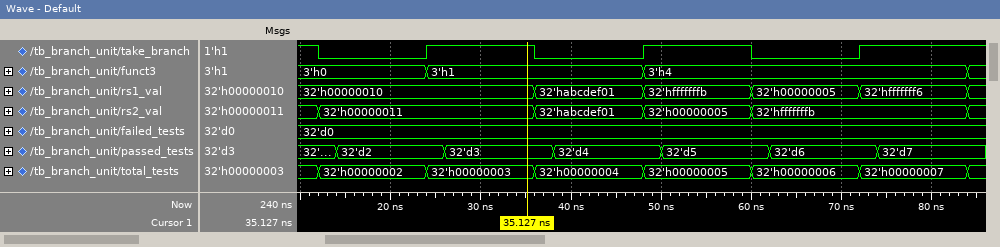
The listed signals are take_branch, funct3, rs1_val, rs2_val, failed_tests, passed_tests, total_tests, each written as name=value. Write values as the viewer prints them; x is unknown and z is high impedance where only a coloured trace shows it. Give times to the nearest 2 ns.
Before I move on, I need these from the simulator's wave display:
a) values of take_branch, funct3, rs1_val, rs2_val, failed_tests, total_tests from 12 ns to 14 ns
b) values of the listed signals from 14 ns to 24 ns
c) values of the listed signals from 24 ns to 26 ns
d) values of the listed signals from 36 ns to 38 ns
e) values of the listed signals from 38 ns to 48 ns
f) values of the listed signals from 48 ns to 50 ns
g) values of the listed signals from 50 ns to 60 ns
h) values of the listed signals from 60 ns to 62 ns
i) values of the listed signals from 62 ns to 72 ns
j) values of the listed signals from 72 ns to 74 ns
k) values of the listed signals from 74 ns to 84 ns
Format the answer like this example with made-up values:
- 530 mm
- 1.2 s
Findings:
- take_branch=0, funct3=3'h0, rs1_val=32'h00000010, rs2_val=32'h00000011, failed_tests=32'd0, total_tests=32'h00000002
- take_branch=0, funct3=3'h0, rs1_val=32'h00000010, rs2_val=32'h00000011, failed_tests=32'd0, passed_tests=32'd2, total_tests=32'h00000002
- take_branch=1, funct3=3'h1, rs1_val=32'h00000010, rs2_val=32'h00000011, failed_tests=32'd0, passed_tests=32'd2, total_tests=32'h00000003
- take_branch=0, funct3=3'h1, rs1_val=32'habcdef01, rs2_val=32'habcdef01, failed_tests=32'd0, passed_tests=32'd3, total_tests=32'h00000004
- take_branch=0, funct3=3'h1, rs1_val=32'habcdef01, rs2_val=32'habcdef01, failed_tests=32'd0, passed_tests=32'd4, total_tests=32'h00000004
- take_branch=1, funct3=3'h4, rs1_val=32'hfffffffb, rs2_val=32'h00000005, failed_tests=32'd0, passed_tests=32'd4, total_tests=32'h00000005
- take_branch=1, funct3=3'h4, rs1_val=32'hfffffffb, rs2_val=32'h00000005, failed_tests=32'd0, passed_tests=32'd5, total_tests=32'h00000005
- take_branch=0, funct3=3'h4, rs1_val=32'h00000005, rs2_val=32'hfffffffb, failed_tests=32'd0, passed_tests=32'd5, total_tests=32'h00000006
- take_branch=0, funct3=3'h4, rs1_val=32'h00000005, rs2_val=32'hfffffffb, failed_tests=32'd0, passed_tests=32'd6, total_tests=32'h00000006
- take_branch=1, funct3=3'h4, rs1_val=32'hfffffff6, rs2_val=32'hfffffffb, failed_tests=32'd0, passed_tests=32'd6, total_tests=32'h00000007
- take_branch=1, funct3=3'h4, rs1_val=32'hfffffff6, rs2_val=32'hfffffffb, failed_tests=32'd0, passed_tests=32'd7, total_tests=32'h00000007
